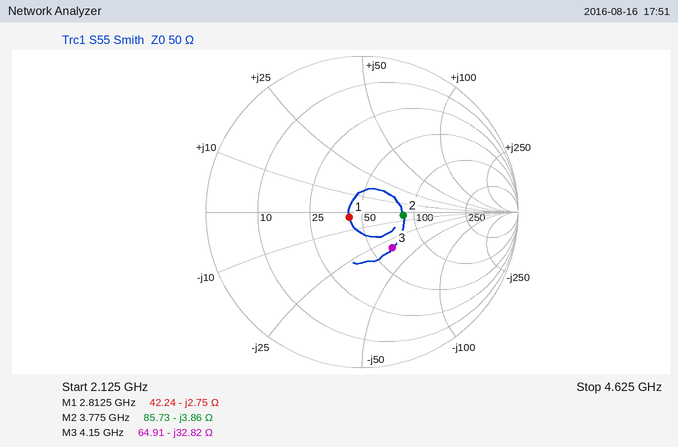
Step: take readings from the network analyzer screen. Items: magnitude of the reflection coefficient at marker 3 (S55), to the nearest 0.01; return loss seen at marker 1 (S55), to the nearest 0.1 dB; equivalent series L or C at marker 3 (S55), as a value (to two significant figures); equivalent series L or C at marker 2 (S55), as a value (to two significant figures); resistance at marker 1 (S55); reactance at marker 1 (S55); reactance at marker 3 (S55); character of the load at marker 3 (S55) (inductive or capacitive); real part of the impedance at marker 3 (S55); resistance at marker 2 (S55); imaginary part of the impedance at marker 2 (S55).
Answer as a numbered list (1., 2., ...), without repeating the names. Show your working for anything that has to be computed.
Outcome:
1. 0.30
2. 21.0 dB
3. C = 1/(2π × 4.15 GHz × 32.82 Ω) ≈ 1.2 pF
4. C = 1/(2π × 3.775 GHz × 3.86 Ω) ≈ 11 pF
5. 42.24 Ω
6. -2.75 Ω
7. -32.82 Ω
8. capacitive
9. 64.91 Ω
10. 85.73 Ω
11. -3.86 Ω
